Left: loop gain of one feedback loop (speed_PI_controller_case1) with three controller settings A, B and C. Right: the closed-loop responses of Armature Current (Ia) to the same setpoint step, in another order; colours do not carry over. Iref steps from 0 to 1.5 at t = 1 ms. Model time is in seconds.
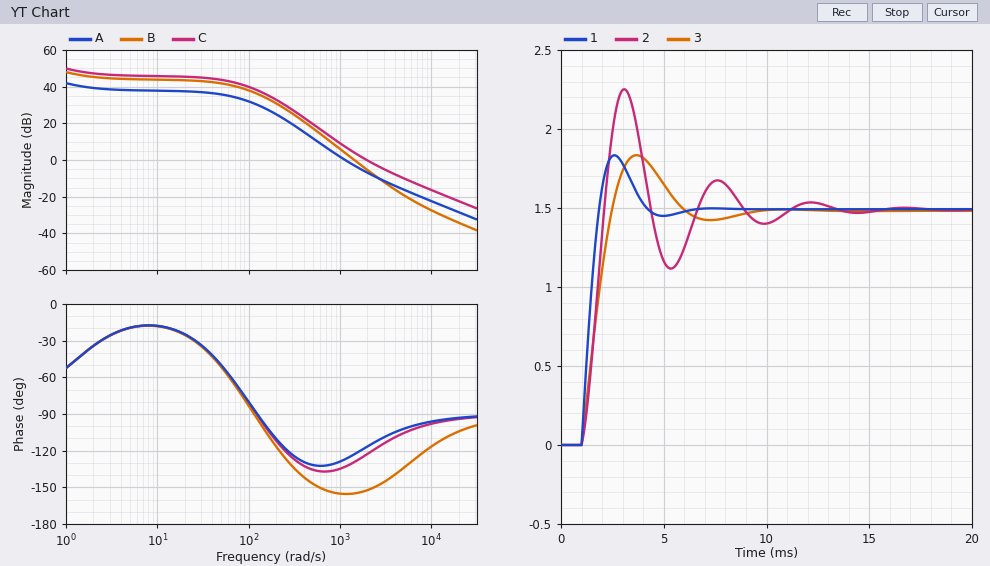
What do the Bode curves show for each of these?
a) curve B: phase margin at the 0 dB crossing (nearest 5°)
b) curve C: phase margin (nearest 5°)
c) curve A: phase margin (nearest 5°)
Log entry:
25°
55°
55°
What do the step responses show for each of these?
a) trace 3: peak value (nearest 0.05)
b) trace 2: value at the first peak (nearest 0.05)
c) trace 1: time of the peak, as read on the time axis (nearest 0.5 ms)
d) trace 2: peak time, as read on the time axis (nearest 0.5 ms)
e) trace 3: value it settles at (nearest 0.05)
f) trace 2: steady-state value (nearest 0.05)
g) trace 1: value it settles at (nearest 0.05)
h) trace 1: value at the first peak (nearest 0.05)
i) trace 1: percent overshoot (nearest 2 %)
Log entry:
1.85
2.25
2.5 ms
3.0 ms
1.50
1.50
1.50
1.85
22 %
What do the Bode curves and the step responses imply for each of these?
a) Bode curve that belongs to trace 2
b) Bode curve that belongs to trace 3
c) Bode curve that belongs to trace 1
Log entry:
B
A
C
